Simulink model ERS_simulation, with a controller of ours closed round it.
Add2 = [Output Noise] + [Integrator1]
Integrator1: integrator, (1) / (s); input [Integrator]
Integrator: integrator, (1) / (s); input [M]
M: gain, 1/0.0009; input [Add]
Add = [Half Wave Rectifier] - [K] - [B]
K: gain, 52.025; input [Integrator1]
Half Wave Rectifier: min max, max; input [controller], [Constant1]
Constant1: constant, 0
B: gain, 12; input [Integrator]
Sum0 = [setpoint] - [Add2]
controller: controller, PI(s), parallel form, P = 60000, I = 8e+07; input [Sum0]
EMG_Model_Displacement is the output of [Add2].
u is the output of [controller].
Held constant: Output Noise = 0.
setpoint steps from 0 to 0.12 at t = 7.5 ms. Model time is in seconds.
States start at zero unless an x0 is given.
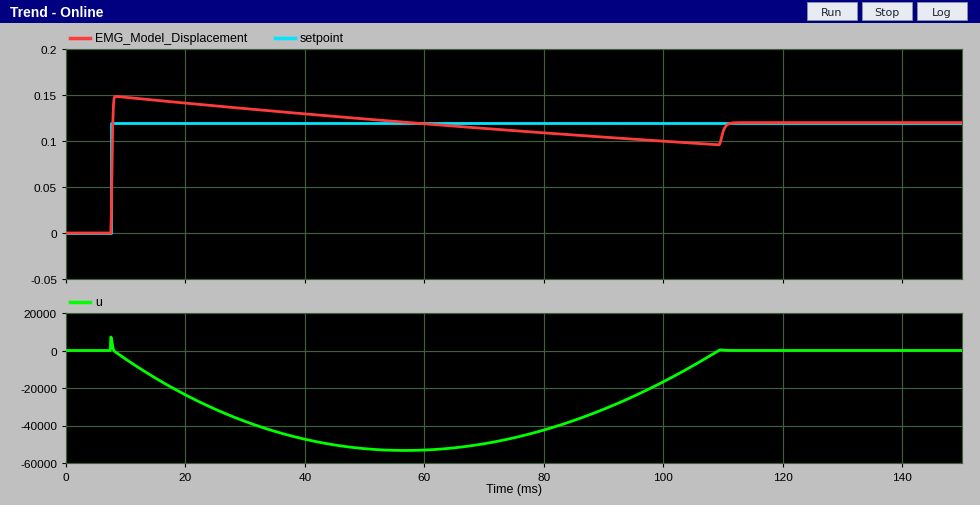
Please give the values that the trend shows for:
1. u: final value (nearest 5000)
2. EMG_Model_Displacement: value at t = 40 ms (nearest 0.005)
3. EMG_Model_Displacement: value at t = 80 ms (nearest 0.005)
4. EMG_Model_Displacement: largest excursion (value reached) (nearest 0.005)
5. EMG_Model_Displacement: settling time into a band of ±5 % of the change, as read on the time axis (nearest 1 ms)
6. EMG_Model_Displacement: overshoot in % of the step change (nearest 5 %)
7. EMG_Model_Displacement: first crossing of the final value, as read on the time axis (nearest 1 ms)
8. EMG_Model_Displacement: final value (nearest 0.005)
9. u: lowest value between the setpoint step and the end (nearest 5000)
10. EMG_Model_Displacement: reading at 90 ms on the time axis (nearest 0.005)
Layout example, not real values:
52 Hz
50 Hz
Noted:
0
0.130
0.110
0.150
110 ms
25 %
8 ms
0.120
-55000
0.105
